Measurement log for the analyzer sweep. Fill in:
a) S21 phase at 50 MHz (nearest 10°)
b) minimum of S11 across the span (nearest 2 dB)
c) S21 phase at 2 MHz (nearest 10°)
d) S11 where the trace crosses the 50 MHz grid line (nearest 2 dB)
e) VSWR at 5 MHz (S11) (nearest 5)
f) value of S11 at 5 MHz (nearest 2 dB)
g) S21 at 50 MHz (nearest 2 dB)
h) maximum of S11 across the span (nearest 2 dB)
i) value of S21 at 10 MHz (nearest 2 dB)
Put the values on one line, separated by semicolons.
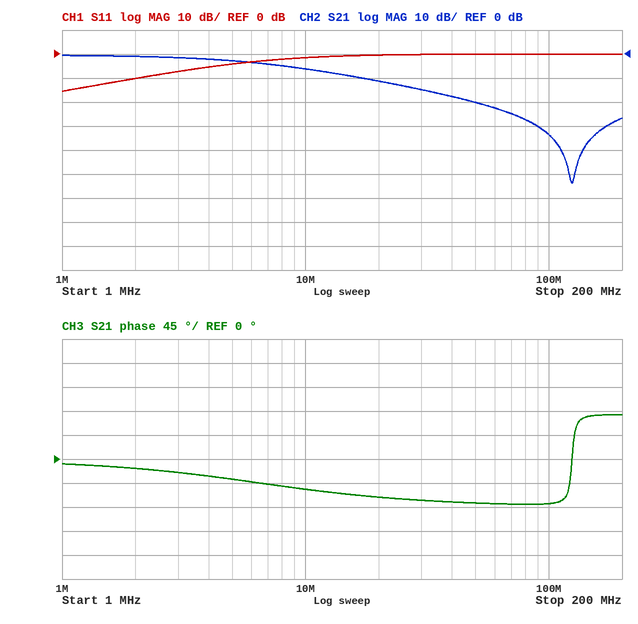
-80°; -16 dB; -20°; 0 dB; 5; -4 dB; -20 dB; 0 dB; -6 dB
